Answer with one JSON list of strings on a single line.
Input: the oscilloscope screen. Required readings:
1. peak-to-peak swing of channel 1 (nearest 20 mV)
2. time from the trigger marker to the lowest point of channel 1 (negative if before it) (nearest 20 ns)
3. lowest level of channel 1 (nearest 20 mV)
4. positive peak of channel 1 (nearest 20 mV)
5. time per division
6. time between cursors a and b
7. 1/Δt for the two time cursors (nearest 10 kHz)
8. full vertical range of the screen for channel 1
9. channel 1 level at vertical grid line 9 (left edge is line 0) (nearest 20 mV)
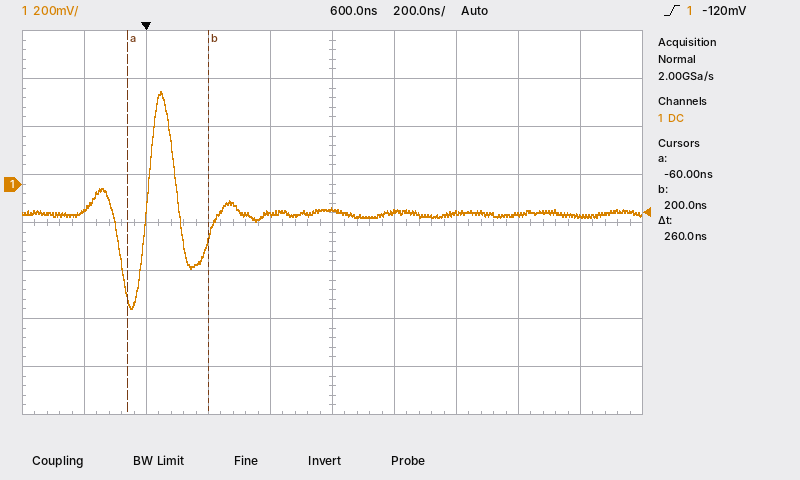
["900 mV", "-40 ns", "-520 mV", "380 mV", "200 ns", "260 ns", "3.85 MHz", "1.6 V", "-140 mV"]
